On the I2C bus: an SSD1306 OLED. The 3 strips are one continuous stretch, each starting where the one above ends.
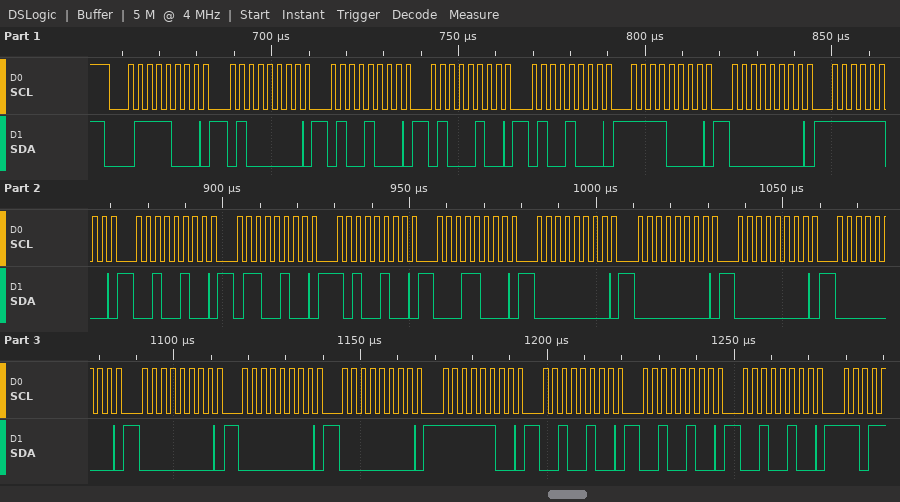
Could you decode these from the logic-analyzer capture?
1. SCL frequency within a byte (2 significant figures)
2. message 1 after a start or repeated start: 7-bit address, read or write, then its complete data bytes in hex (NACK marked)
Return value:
400 kHz
0x3C write: 40 48 44 48 F0 00 FC 24 64 A4 18 00 00 00 00 00 00 00 FC 24 24 24
